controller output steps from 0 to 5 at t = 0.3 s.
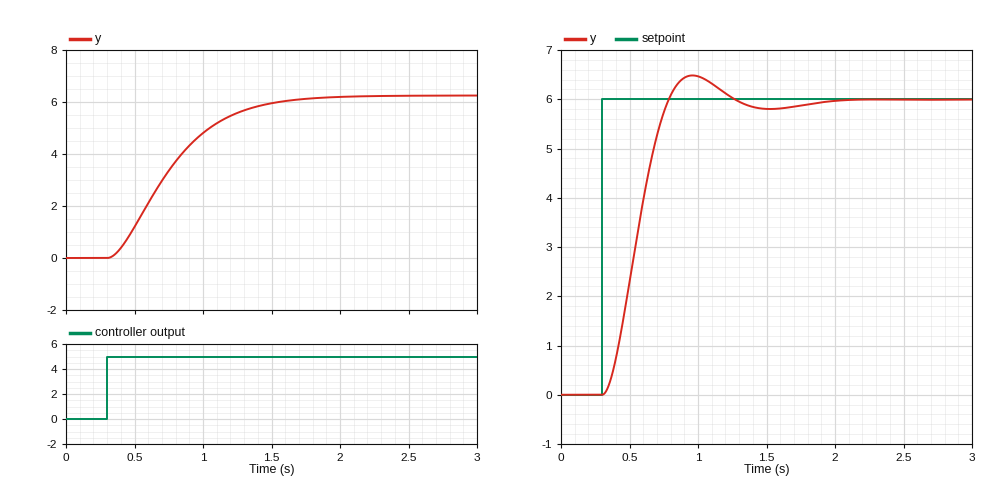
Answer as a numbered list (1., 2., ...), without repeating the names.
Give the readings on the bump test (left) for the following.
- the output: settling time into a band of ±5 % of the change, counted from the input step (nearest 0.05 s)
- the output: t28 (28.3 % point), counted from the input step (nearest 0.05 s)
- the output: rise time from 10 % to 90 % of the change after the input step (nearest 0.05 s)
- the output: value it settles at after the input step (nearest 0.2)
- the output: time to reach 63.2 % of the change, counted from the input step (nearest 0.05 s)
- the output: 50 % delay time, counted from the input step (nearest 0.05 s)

1. 1.20 s
2. 0.25 s
3. 0.85 s
4. 6.2
5. 0.55 s
6. 0.40 s
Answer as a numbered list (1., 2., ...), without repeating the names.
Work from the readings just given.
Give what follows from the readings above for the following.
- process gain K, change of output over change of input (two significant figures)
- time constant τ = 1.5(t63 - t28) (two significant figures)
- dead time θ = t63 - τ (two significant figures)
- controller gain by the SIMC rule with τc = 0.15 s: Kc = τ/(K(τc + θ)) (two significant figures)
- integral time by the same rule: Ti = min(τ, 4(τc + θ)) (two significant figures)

1. 1.2
2. 0.45 s
3. 0.10 s
4. 1.5
5. 0.45 s
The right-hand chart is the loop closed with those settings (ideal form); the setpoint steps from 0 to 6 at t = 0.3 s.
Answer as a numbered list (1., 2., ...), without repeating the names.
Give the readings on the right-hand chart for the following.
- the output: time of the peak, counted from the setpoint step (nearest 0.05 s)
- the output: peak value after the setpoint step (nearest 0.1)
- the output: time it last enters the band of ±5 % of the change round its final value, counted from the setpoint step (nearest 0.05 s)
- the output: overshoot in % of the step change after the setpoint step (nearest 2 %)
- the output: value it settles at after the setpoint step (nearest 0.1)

1. 0.65 s
2. 6.5
3. 0.80 s
4. 8 %
5. 6.0
